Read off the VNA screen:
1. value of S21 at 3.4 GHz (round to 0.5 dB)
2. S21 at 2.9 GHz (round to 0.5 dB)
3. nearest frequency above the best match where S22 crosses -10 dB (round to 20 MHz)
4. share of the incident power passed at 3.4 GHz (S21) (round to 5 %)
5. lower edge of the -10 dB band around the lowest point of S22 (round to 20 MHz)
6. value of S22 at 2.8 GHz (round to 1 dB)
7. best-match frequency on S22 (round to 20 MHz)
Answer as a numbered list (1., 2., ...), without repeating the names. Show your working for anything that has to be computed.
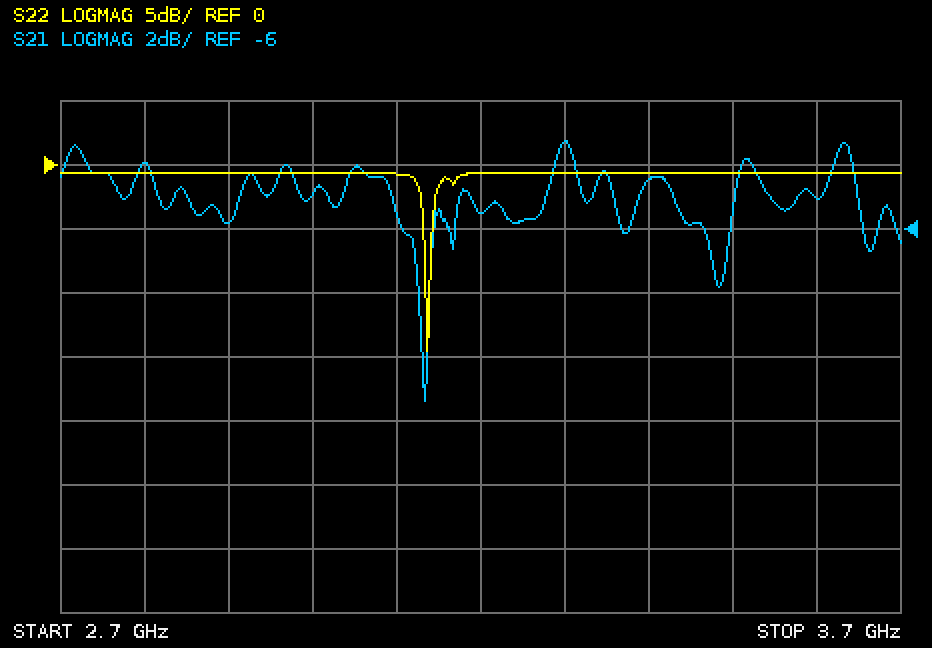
1. -4.5 dB
2. -6.0 dB
3. 3.14 GHz
4. 10^(-4.5/10) ≈ 35 %
5. 3.14 GHz
6. -1 dB
7. 3.14 GHz
